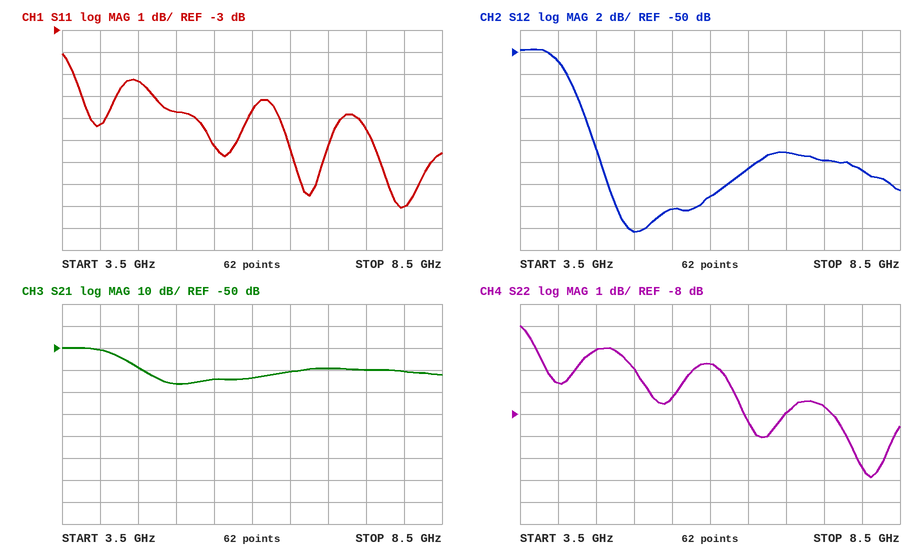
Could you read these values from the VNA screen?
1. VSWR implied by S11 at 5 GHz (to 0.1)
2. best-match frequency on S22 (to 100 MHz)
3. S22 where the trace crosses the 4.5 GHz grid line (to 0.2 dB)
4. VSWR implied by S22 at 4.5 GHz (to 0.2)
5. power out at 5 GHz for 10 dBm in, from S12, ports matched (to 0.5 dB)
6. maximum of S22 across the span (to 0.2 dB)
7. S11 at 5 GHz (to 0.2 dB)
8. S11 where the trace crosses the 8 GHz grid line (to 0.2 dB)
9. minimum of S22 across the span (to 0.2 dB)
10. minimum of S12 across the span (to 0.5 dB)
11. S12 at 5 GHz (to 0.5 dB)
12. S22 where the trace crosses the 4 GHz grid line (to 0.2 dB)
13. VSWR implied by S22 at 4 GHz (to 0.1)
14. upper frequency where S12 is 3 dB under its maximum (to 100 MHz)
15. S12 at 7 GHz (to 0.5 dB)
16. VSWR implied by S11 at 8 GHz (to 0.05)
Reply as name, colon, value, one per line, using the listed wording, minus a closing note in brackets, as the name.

VSWR implied by S11 at 5 GHz: 2.7
best-match frequency on S22: 8.1 GHz
S22 where the trace crosses the 4.5 GHz grid line: -5.0 dB
VSWR implied by S22 at 4.5 GHz: 3.6
power out at 5 GHz for 10 dBm in, from S12, ports matched: -56.5 dBm
maximum of S22 across the span: -4.0 dB
S11 at 5 GHz: -6.8 dB
S11 where the trace crosses the 8 GHz grid line: -11.0 dB
minimum of S22 across the span: -10.8 dB
minimum of S12 across the span: -66.5 dB
S12 at 5 GHz: -66.5 dB
S22 where the trace crosses the 4 GHz grid line: -6.6 dB
VSWR implied by S22 at 4 GHz: 2.8
upper frequency where S12 is 3 dB under its maximum: 4.2 GHz
S12 at 7 GHz: -59.0 dB
VSWR implied by S11 at 8 GHz: 1.80
